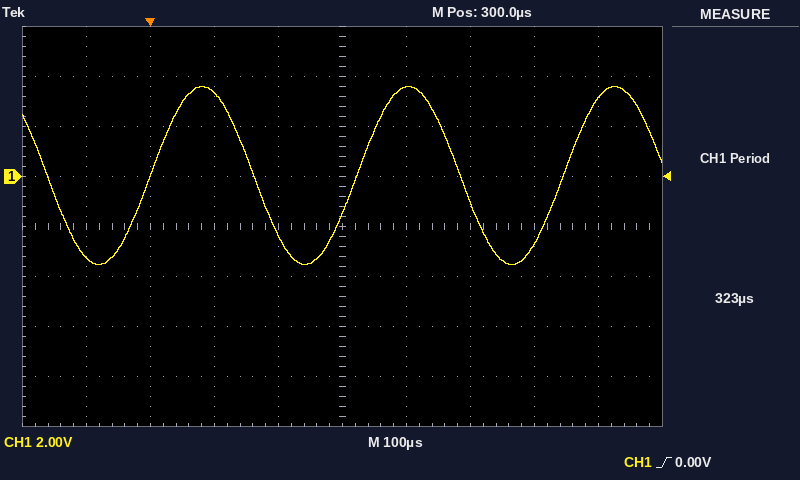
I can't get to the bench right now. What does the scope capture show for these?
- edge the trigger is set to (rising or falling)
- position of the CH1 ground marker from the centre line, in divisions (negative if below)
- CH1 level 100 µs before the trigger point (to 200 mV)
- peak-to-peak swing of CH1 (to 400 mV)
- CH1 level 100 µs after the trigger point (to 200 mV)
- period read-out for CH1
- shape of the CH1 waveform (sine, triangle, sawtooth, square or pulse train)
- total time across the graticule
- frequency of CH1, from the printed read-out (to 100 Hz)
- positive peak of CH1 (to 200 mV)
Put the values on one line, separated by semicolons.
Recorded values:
rising; +1.0 div; -3.2 V; 7.2 V; 3.4 V; 323 µs; sine; 1 ms; 3.1 kHz; 3.6 V
